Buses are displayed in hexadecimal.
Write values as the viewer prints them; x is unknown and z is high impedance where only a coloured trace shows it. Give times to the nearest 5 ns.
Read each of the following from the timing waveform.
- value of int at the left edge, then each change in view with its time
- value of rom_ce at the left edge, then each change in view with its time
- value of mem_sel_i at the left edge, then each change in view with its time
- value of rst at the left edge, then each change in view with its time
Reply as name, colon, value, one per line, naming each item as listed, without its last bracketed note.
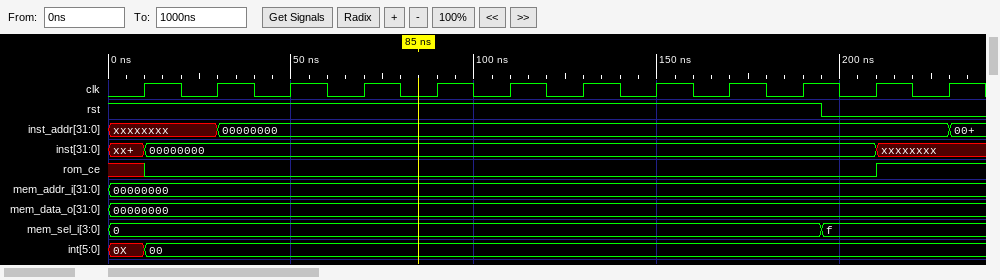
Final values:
value of int at the left edge, then each change in view with its time: 0X, 00 at 10 ns
value of rom_ce at the left edge, then each change in view with its time: x, 0 at 10 ns, 1 at 210 ns
value of mem_sel_i at the left edge, then each change in view with its time: 0, f at 195 ns
value of rst at the left edge, then each change in view with its time: 1, 0 at 195 ns
